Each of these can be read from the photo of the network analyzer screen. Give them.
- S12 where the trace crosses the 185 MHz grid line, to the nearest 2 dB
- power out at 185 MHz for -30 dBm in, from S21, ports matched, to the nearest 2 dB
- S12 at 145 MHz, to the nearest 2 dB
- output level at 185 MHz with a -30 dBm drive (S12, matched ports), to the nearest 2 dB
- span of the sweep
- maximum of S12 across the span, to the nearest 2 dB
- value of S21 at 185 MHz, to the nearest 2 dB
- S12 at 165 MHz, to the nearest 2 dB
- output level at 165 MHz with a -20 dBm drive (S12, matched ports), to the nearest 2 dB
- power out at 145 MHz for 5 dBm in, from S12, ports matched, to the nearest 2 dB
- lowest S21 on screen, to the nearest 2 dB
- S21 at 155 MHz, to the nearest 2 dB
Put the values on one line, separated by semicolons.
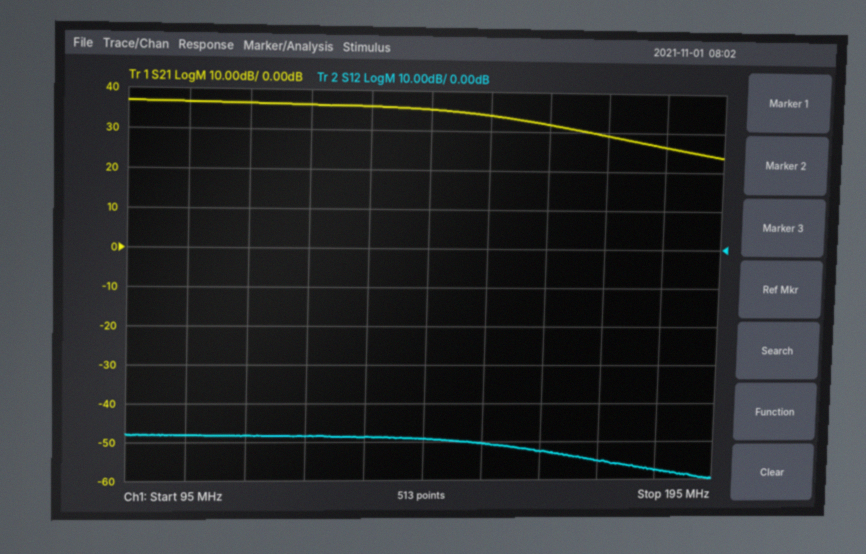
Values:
-58 dB; -4 dBm; -50 dB; -88 dBm; 100 MHz; -48 dB; 26 dB; -52 dB; -72 dBm; -44 dBm; 24 dB; 34 dB
